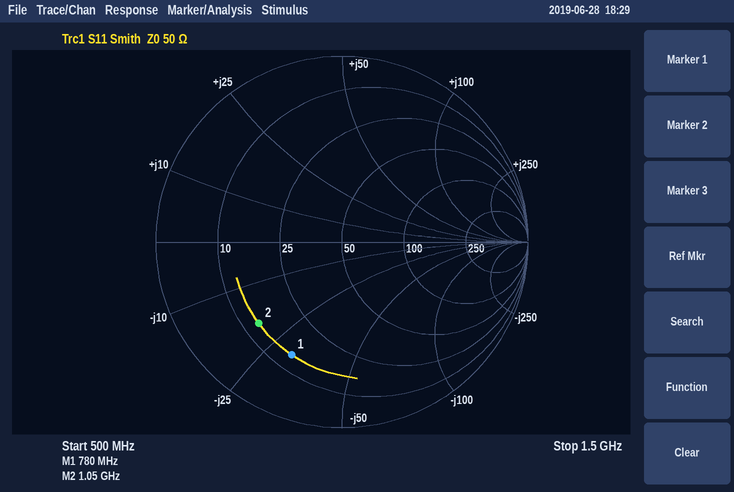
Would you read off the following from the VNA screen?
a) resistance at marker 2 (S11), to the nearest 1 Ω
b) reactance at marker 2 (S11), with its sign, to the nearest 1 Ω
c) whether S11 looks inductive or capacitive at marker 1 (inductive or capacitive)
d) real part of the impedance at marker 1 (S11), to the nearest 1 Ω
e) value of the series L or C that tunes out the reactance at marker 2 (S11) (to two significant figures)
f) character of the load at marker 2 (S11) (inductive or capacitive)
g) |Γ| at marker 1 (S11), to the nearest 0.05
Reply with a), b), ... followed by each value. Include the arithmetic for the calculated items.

a) 13 Ω
b) -19 Ω
c) capacitive
d) 14 Ω
e) L = 19 Ω/(2π × 1.05 GHz) ≈ 2.9 nH
f) capacitive
g) 0.65
